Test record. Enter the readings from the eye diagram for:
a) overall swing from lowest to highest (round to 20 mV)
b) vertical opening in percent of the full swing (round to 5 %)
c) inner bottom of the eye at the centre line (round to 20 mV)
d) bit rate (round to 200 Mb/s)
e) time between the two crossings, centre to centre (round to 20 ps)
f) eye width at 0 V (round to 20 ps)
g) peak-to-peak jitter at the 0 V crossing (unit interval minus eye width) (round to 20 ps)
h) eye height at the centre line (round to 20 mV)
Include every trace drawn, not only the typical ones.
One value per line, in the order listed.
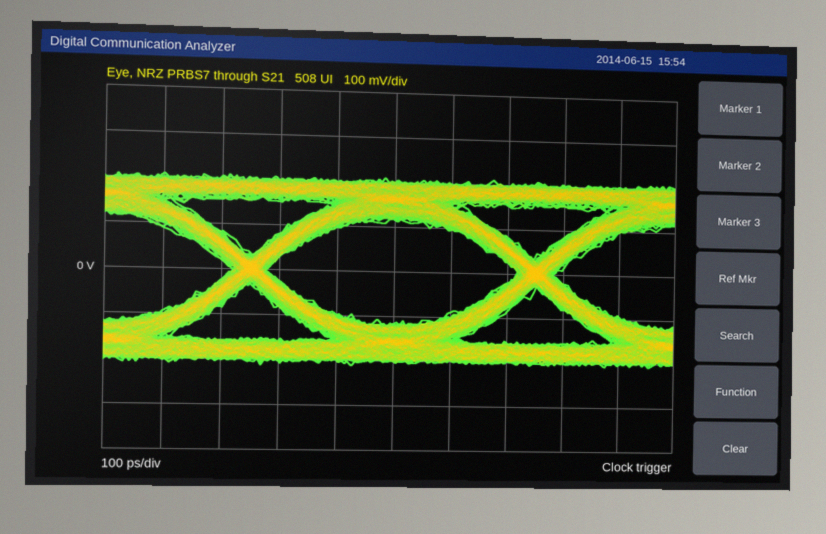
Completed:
420 mV
55 %
-120 mV
2.0 Gb/s
500 ps
440 ps
60 ps
240 mV
